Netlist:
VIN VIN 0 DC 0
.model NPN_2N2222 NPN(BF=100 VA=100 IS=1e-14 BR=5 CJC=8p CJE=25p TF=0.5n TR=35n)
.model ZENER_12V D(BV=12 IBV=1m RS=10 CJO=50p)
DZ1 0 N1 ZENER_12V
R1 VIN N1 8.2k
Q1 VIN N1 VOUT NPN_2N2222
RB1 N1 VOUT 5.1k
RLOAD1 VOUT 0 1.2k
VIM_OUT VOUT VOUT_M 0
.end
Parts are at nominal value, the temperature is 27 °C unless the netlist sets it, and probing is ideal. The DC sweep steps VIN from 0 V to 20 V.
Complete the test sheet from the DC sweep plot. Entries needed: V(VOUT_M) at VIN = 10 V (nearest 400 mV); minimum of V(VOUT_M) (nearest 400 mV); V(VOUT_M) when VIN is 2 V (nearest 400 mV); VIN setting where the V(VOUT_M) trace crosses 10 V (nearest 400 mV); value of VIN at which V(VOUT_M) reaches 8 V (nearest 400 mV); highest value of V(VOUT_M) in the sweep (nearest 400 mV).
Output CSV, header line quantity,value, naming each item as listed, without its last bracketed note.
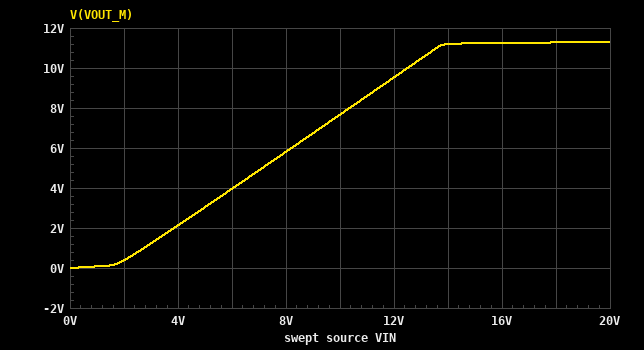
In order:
quantity,value
V(VOUT_M) at VIN = 10 V,7.6 V
minimum of V(VOUT_M),0 V
V(VOUT_M) when VIN is 2 V,400 mV
VIN setting where the V(VOUT_M) trace crosses 10 V,12.4 V
value of VIN at which V(VOUT_M) reaches 8 V,10.4 V
highest value of V(VOUT_M) in the sweep,11.2 V
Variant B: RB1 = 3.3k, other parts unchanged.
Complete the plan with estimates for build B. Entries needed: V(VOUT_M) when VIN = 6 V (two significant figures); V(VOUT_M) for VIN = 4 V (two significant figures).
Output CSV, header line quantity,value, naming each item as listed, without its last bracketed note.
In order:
quantity,value
V(VOUT_M) when VIN = 6 V,3.4 V
V(VOUT_M) for VIN = 4 V,1.6 V
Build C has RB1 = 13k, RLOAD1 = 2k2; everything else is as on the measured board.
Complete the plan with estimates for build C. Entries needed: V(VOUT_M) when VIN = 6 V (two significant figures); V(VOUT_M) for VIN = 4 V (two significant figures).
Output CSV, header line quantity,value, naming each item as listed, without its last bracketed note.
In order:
quantity,value
V(VOUT_M) when VIN = 6 V,4.7 V
V(VOUT_M) for VIN = 4 V,2.8 V
